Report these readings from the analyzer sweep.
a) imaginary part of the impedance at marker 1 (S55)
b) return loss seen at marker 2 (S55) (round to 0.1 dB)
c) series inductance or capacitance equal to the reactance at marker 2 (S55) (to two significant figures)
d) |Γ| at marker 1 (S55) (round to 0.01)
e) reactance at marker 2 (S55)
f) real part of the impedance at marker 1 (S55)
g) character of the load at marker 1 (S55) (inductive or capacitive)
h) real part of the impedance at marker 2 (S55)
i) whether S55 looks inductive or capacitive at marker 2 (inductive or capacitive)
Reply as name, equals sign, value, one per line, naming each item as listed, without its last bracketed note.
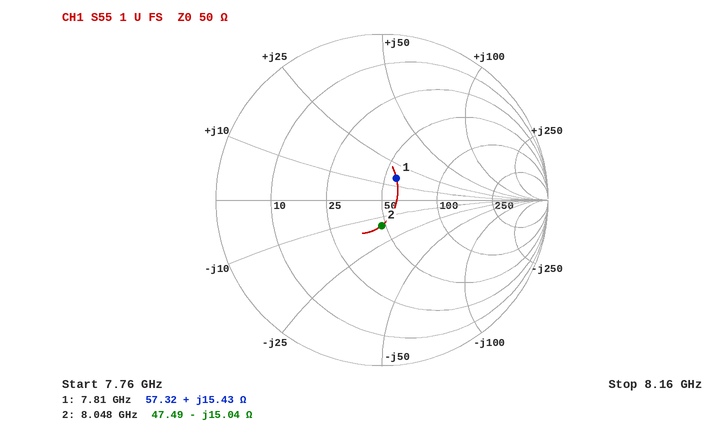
imaginary part of the impedance at marker 1 = +15.43 Ω
return loss seen at marker 2 (S55) = 16.2 dB
series inductance or capacitance equal to the reactance at marker 2 (S55) = 1.3 pF
|Γ| at marker 1 (S55) = 0.16
reactance at marker 2 = -15.04 Ω
real part of the impedance at marker 1 = 57.32 Ω
character of the load at marker 1 (S55) = inductive
real part of the impedance at marker 2 = 47.49 Ω
whether S55 looks inductive or capacitive at marker 2 = capacitive
